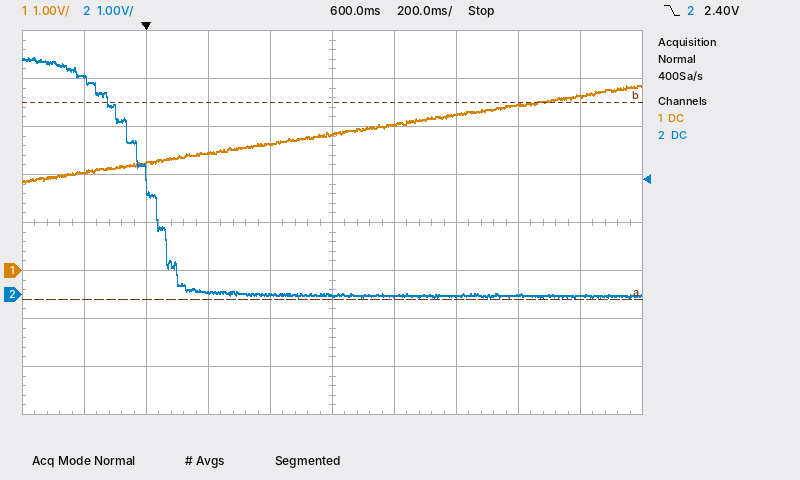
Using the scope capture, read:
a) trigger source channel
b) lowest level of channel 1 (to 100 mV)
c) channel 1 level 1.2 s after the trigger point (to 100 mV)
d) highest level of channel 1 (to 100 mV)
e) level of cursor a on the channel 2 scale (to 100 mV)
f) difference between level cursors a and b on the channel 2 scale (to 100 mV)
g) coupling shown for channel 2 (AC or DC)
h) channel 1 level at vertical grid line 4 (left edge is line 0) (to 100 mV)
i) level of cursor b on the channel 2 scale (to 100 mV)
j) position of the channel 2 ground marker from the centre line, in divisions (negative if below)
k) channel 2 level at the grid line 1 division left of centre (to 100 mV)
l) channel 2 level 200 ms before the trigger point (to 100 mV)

channel 2
1.8 V
3.5 V
3.9 V
-100 mV
4.1 V
DC
2.6 V
4.0 V
-1.5 div
0.0 V
4.5 V
